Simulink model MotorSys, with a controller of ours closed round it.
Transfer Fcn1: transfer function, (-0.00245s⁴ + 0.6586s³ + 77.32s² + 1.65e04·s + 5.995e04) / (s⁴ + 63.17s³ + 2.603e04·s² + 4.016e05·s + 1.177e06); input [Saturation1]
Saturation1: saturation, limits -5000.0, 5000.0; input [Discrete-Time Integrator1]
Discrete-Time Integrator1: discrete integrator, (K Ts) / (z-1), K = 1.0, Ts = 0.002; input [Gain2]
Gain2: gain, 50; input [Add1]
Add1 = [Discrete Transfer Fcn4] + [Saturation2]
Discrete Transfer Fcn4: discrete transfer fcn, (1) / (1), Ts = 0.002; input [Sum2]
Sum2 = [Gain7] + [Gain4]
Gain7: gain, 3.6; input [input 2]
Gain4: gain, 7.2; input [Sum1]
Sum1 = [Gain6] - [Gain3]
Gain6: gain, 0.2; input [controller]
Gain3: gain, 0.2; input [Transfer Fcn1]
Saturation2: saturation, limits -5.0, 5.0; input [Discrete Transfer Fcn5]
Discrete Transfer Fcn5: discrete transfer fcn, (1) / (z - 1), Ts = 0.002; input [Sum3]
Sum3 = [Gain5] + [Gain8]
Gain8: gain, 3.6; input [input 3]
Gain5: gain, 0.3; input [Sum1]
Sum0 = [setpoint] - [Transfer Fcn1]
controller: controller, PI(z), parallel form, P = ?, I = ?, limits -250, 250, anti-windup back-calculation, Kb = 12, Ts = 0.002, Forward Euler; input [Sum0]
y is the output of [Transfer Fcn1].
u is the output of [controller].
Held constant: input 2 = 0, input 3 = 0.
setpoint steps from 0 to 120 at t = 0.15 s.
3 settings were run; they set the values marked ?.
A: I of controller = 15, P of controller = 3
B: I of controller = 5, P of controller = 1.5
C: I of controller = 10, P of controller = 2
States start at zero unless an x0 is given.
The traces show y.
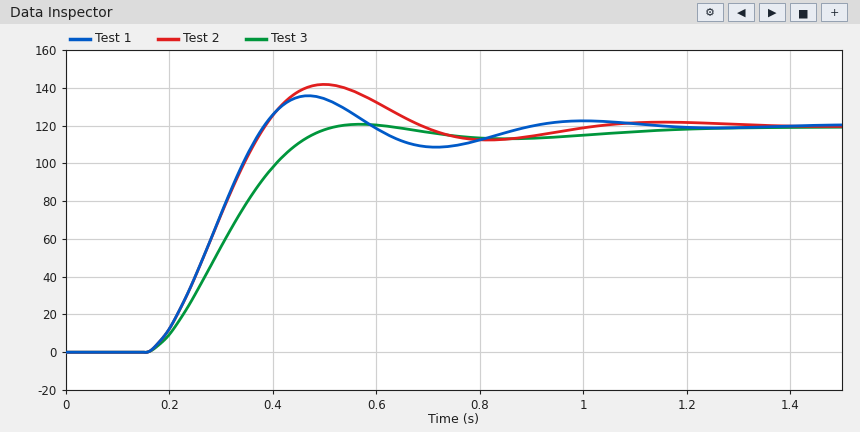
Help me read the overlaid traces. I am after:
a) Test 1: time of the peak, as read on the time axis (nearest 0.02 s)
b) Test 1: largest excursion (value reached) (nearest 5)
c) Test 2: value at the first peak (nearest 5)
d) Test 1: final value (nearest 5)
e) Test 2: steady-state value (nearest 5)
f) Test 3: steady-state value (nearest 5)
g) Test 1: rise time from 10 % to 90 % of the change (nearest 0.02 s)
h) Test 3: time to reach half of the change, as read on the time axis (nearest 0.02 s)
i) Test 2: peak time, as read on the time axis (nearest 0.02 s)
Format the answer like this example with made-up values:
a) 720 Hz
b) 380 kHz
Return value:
a) 0.46 s
b) 135
c) 140
d) 120
e) 120
f) 120
g) 0.16 s
h) 0.30 s
i) 0.50 s
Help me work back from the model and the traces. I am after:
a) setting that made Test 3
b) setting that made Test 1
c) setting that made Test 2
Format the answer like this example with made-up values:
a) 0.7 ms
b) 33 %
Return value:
a) B
b) A
c) C
